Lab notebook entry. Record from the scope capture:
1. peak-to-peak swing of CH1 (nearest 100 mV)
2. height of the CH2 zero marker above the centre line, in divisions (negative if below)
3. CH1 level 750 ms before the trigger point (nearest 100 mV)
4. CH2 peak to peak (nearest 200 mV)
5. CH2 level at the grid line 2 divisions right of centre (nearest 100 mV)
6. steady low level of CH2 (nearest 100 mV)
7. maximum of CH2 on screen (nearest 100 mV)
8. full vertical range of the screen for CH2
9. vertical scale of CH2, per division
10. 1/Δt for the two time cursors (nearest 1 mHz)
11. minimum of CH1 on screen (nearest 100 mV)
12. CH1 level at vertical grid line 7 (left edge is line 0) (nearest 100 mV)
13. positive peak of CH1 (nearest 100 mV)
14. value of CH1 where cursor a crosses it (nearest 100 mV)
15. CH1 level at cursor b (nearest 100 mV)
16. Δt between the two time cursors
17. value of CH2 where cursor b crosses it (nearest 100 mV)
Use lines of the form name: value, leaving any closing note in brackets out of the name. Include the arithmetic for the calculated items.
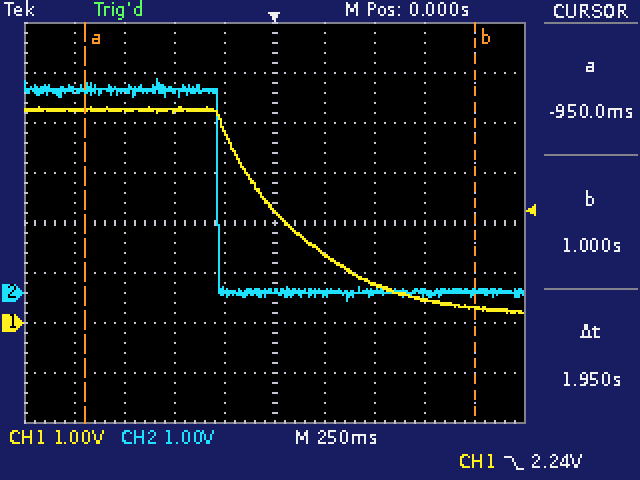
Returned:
peak-to-peak swing of CH1: 4.3 V − (200 mV) = 4.1 V
height of the CH2 zero marker above the centre line, in divisions: -1.4 div
CH1 level 750 ms before the trigger point: 4.3 V
CH2 peak to peak: 4.4 V
CH2 level at the grid line 2 divisions right of centre: 0.0 V
steady low level of CH2: 0.0 V
maximum of CH2 on screen: 4.3 V
full vertical range of the screen for CH2: 8 V
vertical scale of CH2, per division: 1 V
1/Δt for the two time cursors: 1 / 1.95 s ≈ 513 mHz
minimum of CH1 on screen: 200 mV
CH1 level at vertical grid line 7 (left edge is line 0): 800 mV
positive peak of CH1: 4.3 V
value of CH1 where cursor a crosses it: 4.3 V
CH1 level at cursor b: 300 mV
Δt between the two time cursors: 1.95 s
value of CH2 where cursor b crosses it: 0.0 V
